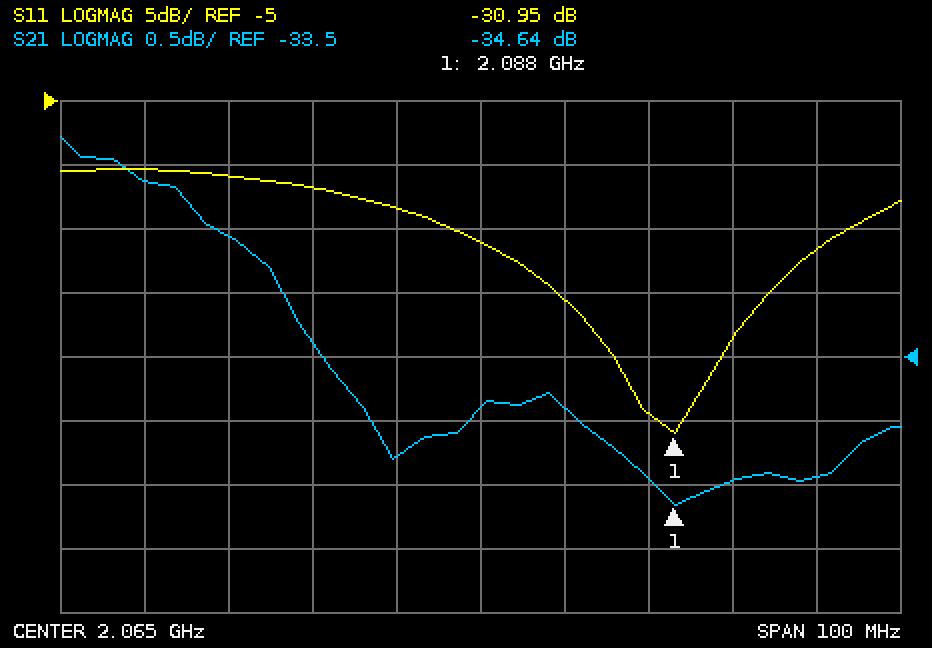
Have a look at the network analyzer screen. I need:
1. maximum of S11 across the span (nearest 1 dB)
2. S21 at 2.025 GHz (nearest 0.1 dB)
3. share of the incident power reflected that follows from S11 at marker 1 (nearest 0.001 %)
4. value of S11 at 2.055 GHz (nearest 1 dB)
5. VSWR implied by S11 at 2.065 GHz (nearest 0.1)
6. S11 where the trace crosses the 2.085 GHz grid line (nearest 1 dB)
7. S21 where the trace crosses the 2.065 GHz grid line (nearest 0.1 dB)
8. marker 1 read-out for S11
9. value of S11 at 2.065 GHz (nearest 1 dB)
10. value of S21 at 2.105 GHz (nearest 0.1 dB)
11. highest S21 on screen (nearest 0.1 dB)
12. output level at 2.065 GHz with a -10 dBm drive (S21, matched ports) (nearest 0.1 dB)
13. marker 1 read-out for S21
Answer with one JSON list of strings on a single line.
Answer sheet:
["-10 dB", "-32.1 dB", "0.080 %", "-13 dB", "1.4", "-29 dB", "-33.9 dB", "-30.95 dB", "-16 dB", "-34.4 dB", "-31.8 dB", "-43.9 dBm", "-34.64 dB"]
